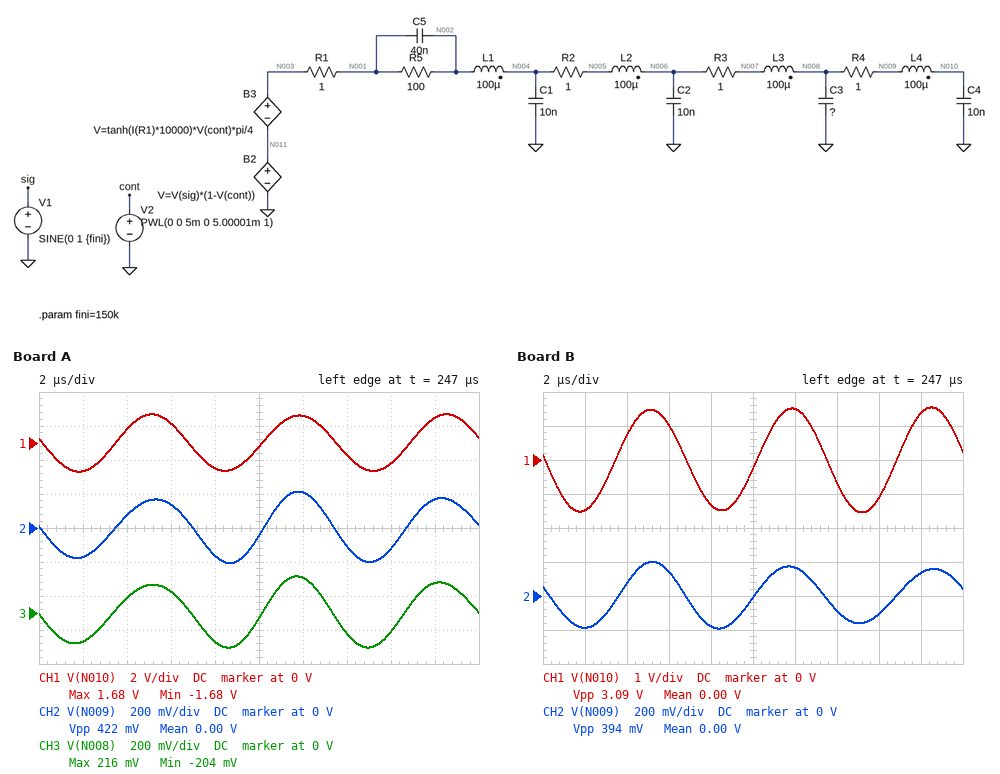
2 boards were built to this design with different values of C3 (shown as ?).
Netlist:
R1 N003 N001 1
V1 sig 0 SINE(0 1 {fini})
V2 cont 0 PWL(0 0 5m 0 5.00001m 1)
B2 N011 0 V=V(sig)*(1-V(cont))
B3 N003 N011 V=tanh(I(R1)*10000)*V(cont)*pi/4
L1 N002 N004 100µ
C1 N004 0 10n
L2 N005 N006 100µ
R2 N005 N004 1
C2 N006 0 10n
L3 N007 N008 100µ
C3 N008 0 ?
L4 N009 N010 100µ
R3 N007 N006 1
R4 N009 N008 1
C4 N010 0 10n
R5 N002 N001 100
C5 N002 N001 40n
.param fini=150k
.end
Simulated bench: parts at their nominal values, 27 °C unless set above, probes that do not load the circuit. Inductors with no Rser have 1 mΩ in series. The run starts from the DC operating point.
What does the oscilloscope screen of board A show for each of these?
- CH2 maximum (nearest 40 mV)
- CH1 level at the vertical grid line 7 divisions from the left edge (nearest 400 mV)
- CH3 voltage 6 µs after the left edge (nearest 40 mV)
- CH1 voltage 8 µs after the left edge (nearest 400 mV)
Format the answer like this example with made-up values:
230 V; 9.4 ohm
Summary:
200 mV; -800 mV; 120 mV; -1.6 V
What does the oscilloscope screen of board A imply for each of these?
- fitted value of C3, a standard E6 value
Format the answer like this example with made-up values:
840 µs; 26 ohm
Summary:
22 nF
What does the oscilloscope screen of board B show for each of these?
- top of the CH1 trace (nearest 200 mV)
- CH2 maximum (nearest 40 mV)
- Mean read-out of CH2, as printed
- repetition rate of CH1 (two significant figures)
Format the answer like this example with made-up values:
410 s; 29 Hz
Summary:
1.6 V; 200 mV; 0.00 V; 150 kHz
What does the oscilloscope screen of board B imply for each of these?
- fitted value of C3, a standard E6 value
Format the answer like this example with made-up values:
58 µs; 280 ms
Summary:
33 nF
